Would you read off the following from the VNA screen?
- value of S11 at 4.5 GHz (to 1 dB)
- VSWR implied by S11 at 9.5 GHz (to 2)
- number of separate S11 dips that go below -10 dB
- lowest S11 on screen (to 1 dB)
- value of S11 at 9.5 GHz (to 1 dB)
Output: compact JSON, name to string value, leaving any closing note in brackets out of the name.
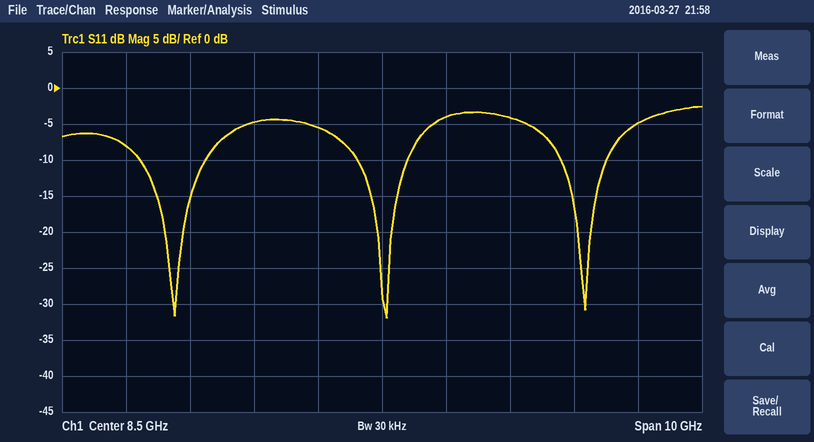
{"value of S11 at 4.5 GHz": "-8 dB", "VSWR implied by S11 at 9.5 GHz": "4", "number of separate S11 dips that go below -10 dB": "3", "lowest S11 on screen": "-32 dB", "value of S11 at 9.5 GHz": "-4 dB"}
